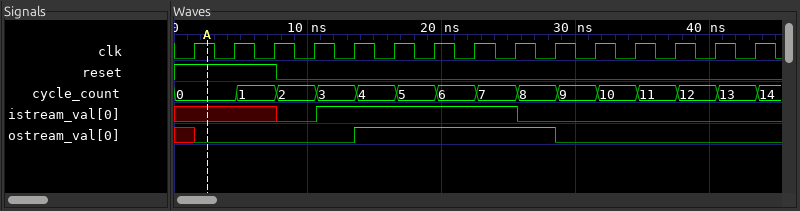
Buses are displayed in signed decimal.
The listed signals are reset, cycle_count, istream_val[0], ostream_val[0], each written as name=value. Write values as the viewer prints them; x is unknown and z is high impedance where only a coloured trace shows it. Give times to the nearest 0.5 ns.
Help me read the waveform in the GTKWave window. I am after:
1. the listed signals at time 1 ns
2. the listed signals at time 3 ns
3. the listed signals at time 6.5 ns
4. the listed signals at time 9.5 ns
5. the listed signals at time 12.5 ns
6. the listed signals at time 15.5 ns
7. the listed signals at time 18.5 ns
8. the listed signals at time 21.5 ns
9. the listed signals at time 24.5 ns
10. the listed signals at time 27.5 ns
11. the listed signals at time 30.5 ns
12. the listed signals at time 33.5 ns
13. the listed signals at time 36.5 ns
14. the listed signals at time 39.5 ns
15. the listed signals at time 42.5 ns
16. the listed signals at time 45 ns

reset=1, cycle_count=0, istream_val[0]=x, ostream_val[0]=x
reset=1, cycle_count=0, istream_val[0]=x, ostream_val[0]=0
reset=1, cycle_count=1, istream_val[0]=x, ostream_val[0]=0
reset=0, cycle_count=2, istream_val[0]=0, ostream_val[0]=0
reset=0, cycle_count=3, istream_val[0]=1, ostream_val[0]=0
reset=0, cycle_count=4, istream_val[0]=1, ostream_val[0]=1
reset=0, cycle_count=5, istream_val[0]=1, ostream_val[0]=1
reset=0, cycle_count=6, istream_val[0]=1, ostream_val[0]=1
reset=0, cycle_count=7, istream_val[0]=1, ostream_val[0]=1
reset=0, cycle_count=8, istream_val[0]=0, ostream_val[0]=1
reset=0, cycle_count=9, istream_val[0]=0, ostream_val[0]=0
reset=0, cycle_count=10, istream_val[0]=0, ostream_val[0]=0
reset=0, cycle_count=11, istream_val[0]=0, ostream_val[0]=0
reset=0, cycle_count=12, istream_val[0]=0, ostream_val[0]=0
reset=0, cycle_count=13, istream_val[0]=0, ostream_val[0]=0
reset=0, cycle_count=14, istream_val[0]=0, ostream_val[0]=0
